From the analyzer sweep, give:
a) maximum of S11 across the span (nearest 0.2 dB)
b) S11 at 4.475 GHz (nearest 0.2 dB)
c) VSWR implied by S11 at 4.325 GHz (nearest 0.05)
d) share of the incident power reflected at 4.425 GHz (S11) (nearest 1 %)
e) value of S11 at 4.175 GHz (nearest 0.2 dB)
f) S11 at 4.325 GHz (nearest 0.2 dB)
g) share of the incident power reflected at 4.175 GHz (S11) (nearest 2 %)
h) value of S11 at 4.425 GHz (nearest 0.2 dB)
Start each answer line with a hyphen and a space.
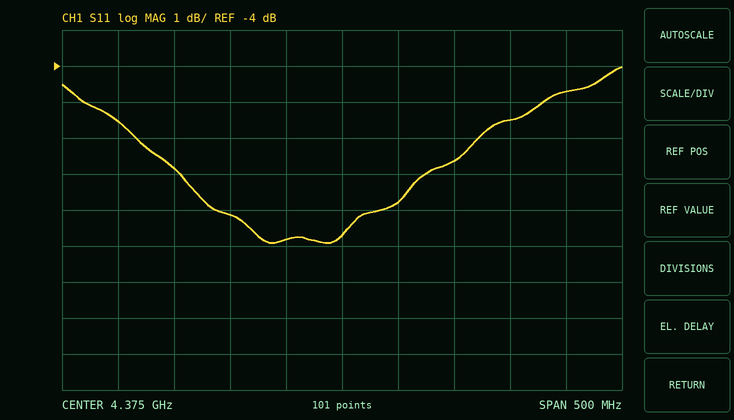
- -4.0 dB
- -6.6 dB
- 2.15
- 17 %
- -5.6 dB
- -8.8 dB
- 28 %
- -7.8 dB
